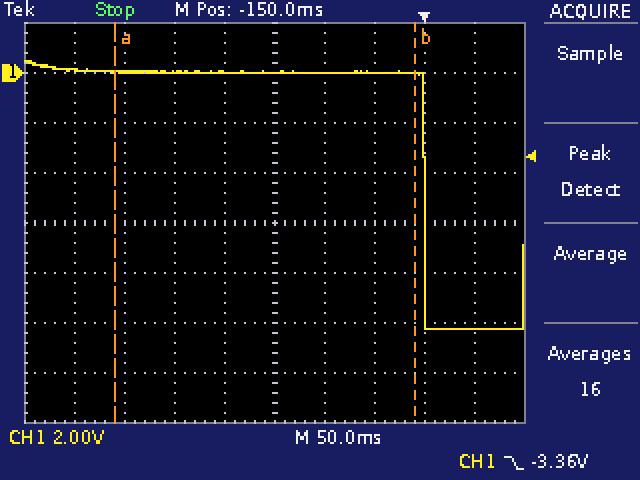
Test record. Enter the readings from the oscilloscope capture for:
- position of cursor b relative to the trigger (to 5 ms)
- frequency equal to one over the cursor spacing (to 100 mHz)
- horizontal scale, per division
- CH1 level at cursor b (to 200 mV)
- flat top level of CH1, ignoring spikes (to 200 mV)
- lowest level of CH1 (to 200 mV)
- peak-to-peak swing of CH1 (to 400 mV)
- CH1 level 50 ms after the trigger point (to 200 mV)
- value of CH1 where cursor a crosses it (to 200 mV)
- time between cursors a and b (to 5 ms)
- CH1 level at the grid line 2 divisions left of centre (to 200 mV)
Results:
-10 ms
3.3 Hz
50 ms
0.0 V
0.0 V
-10.2 V
10.8 V
-10.2 V
0.0 V
300 ms
0.0 V
